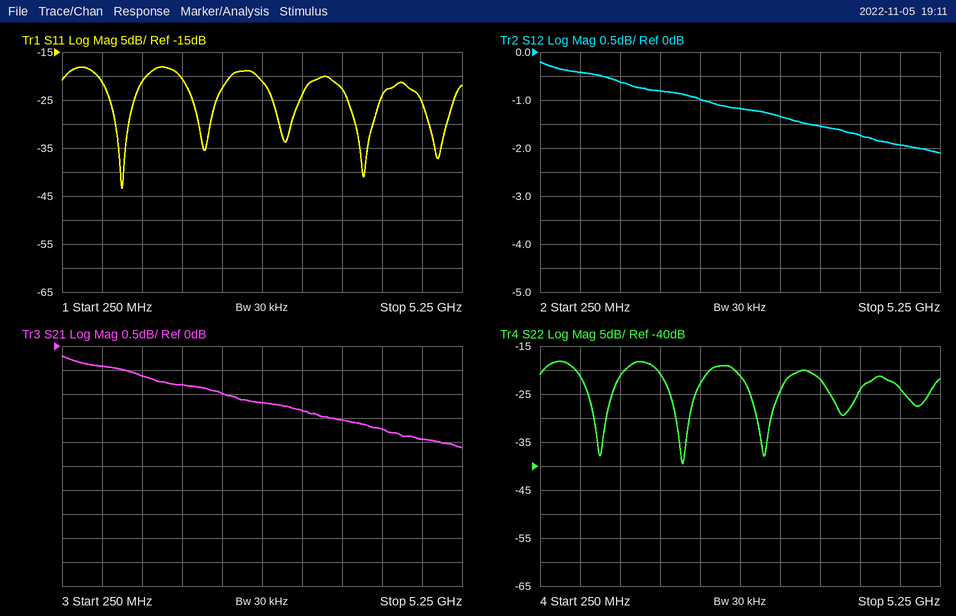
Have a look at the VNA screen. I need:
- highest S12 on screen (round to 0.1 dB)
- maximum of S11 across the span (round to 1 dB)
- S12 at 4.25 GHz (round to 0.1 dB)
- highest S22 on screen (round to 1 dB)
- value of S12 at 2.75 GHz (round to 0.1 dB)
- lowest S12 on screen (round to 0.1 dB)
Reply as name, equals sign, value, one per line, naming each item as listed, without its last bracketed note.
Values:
highest S12 on screen = -0.2 dB
maximum of S11 across the span = -18 dB
S12 at 4.25 GHz = -1.7 dB
highest S22 on screen = -18 dB
value of S12 at 2.75 GHz = -1.2 dB
lowest S12 on screen = -2.1 dB
